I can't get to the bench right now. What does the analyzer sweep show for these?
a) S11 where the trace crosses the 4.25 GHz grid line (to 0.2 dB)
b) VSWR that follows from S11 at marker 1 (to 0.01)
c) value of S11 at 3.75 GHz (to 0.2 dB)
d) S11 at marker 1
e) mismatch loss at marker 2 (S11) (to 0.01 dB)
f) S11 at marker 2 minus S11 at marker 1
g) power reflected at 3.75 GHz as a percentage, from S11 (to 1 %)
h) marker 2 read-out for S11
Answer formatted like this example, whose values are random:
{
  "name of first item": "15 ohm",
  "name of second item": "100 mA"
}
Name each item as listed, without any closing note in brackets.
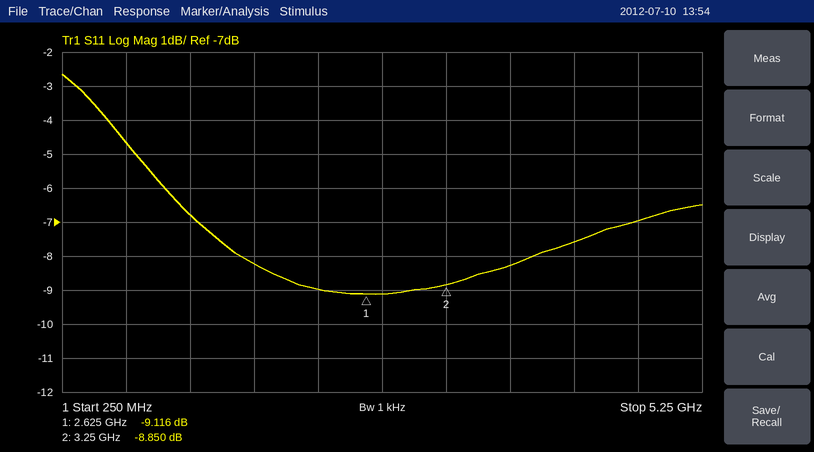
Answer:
{
  "S11 where the trace crosses the 4.25 GHz grid line": "-7.6 dB",
  "VSWR that follows from S11 at marker 1": "2.08",
  "value of S11 at 3.75 GHz": "-8.2 dB",
  "S11 at marker 1": "-9.116 dB",
  "mismatch loss at marker 2 (S11)": "0.61 dB",
  "S11 at marker 2 minus S11 at marker 1": "0.266 dB",
  "power reflected at 3.75 GHz as a percentage, from S11": "15 %",
  "marker 2 read-out for S11": "-8.850 dB"
}
